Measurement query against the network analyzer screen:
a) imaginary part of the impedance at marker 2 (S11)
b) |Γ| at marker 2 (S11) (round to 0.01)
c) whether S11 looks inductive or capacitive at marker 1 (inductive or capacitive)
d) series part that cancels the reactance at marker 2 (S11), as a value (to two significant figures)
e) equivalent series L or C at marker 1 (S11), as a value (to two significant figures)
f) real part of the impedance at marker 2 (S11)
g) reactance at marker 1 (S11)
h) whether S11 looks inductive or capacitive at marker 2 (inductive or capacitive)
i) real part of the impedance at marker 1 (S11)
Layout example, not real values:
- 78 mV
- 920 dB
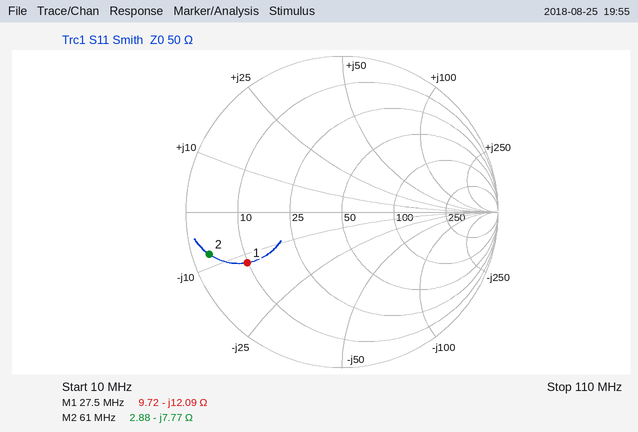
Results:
- -7.77 Ω
- 0.89
- capacitive
- 20 nH
- 480 pF
- 2.88 Ω
- -12.09 Ω
- capacitive
- 9.72 Ω
